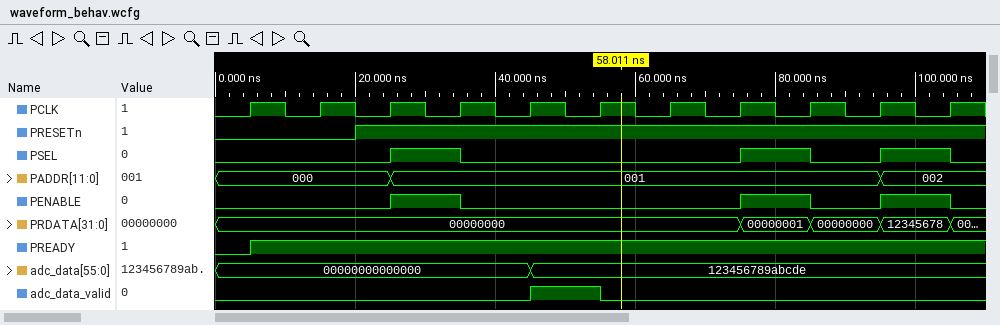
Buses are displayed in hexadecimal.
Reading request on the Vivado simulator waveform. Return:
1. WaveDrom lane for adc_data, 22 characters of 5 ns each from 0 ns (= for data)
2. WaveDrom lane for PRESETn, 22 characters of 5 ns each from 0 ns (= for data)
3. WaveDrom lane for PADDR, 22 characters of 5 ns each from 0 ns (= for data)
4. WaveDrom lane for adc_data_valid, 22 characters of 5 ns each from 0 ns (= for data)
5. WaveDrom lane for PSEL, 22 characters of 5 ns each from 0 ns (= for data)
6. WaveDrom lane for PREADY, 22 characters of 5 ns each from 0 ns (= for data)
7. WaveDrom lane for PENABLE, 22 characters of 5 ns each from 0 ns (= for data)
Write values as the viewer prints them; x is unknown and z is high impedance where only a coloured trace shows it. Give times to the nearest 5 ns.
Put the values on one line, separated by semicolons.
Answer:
{name: 'adc_data', wave: '=........=............', data: '00000000000000 123456789abcde'}; {name: 'PRESETn', wave: '0...1.................'}; {name: 'PADDR', wave: '=....=.............=..', data: '000 001 002'}; {name: 'adc_data_valid', wave: '0........1.0..........'}; {name: 'PSEL', wave: '0....1.0.......1.0.1.0'}; {name: 'PREADY', wave: '01....................'}; {name: 'PENABLE', wave: '0....1.0.......1.0.1.0'}
